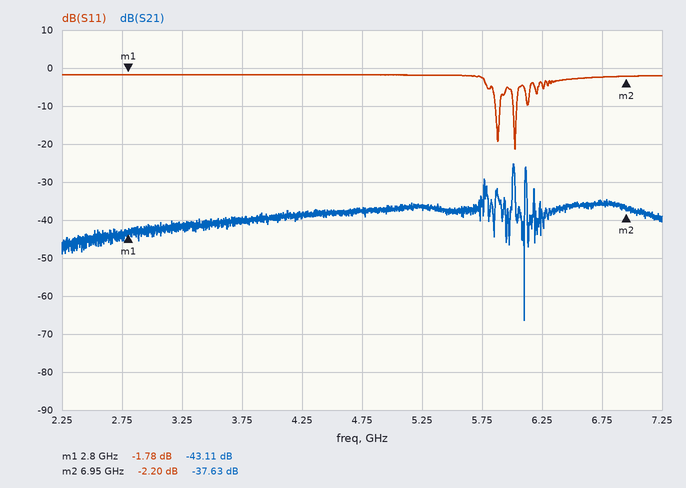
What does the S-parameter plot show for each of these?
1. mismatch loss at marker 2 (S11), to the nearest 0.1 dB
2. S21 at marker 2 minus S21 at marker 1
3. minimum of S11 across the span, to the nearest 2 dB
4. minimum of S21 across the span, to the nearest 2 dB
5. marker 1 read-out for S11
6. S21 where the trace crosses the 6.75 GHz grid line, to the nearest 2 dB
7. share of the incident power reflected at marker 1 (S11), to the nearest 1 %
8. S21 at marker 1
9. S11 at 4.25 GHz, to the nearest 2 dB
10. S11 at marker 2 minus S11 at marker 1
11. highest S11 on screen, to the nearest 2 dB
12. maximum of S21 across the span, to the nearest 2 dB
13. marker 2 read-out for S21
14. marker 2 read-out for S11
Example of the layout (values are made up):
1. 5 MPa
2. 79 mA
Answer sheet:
1. 4.0 dB
2. 5.48 dB
3. -22 dB
4. -66 dB
5. -1.78 dB
6. -36 dB
7. 66 %
8. -43.11 dB
9. -2 dB
10. -0.42 dB
11. -2 dB
12. -26 dB
13. -37.63 dB
14. -2.20 dB
